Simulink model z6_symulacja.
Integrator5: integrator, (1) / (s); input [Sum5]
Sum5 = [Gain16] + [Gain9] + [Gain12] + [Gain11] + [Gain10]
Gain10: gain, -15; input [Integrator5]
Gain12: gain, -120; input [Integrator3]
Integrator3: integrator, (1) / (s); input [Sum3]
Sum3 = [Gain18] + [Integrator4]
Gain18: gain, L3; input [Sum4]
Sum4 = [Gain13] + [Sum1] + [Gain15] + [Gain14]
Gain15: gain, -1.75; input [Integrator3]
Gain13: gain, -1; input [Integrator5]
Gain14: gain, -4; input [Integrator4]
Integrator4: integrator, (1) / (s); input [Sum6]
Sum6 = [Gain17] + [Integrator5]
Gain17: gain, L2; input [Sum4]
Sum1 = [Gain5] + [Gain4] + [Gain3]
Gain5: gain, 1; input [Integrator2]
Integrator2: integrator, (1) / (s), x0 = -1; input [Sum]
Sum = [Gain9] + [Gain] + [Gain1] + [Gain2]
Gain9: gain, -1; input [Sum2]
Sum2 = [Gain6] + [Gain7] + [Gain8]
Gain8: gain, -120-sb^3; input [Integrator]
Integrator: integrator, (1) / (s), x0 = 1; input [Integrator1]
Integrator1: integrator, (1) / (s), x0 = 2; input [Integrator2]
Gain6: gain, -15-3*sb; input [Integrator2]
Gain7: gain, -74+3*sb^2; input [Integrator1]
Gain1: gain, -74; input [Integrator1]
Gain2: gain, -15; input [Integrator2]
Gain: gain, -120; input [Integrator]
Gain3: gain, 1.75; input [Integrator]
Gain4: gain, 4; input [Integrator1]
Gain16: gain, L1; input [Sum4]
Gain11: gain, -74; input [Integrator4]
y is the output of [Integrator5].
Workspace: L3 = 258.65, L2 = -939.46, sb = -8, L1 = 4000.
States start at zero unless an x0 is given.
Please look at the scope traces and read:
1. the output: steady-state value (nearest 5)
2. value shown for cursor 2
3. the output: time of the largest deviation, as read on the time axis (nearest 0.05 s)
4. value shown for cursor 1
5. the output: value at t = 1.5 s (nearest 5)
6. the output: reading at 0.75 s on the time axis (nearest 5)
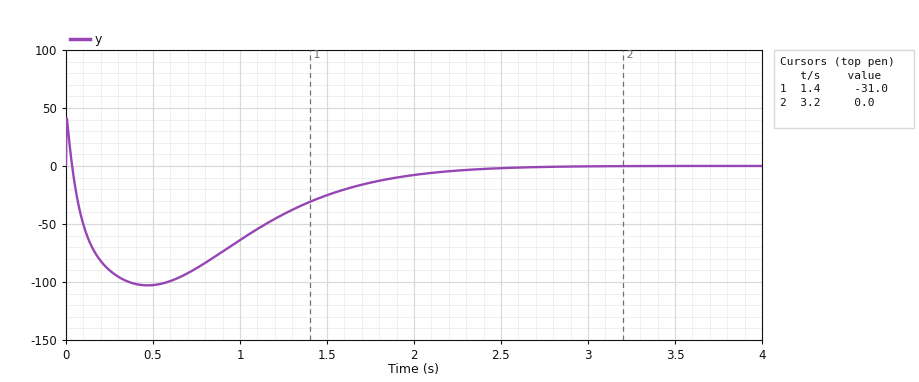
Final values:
0
0.0
0.45 s
-31.0
-25
-90
